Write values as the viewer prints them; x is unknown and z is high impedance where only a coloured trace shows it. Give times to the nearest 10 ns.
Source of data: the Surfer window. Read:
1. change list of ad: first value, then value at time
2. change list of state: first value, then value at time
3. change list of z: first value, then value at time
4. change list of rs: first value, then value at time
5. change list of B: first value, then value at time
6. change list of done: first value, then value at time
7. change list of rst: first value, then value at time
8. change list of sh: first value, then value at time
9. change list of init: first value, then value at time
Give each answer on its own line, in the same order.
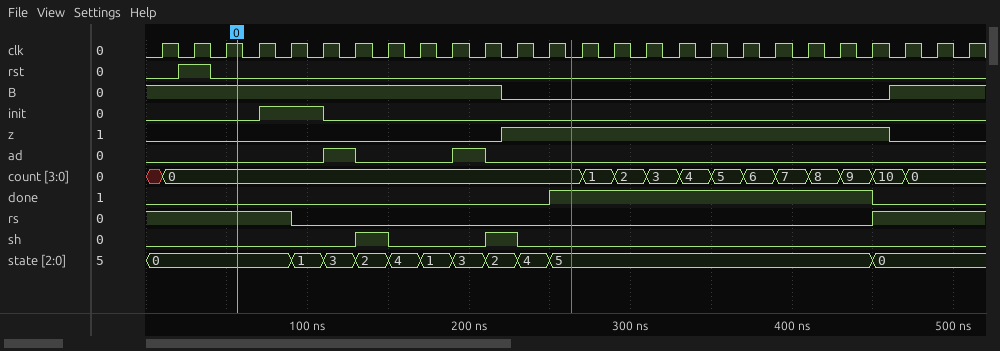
0, 1 at 110 ns, 0 at 130 ns, 1 at 190 ns, 0 at 210 ns
0, 1 at 90 ns, 3 at 110 ns, 2 at 130 ns, 4 at 150 ns, 1 at 170 ns, 3 at 190 ns, 2 at 210 ns, 4 at 230 ns, 5 at 250 ns, 0 at 450 ns
0, 1 at 220 ns, 0 at 460 ns
1, 0 at 90 ns, 1 at 450 ns
1, 0 at 220 ns, 1 at 460 ns
0, 1 at 250 ns, 0 at 450 ns
0, 1 at 20 ns, 0 at 40 ns
0, 1 at 130 ns, 0 at 150 ns, 1 at 210 ns, 0 at 230 ns
0, 1 at 70 ns, 0 at 110 ns
